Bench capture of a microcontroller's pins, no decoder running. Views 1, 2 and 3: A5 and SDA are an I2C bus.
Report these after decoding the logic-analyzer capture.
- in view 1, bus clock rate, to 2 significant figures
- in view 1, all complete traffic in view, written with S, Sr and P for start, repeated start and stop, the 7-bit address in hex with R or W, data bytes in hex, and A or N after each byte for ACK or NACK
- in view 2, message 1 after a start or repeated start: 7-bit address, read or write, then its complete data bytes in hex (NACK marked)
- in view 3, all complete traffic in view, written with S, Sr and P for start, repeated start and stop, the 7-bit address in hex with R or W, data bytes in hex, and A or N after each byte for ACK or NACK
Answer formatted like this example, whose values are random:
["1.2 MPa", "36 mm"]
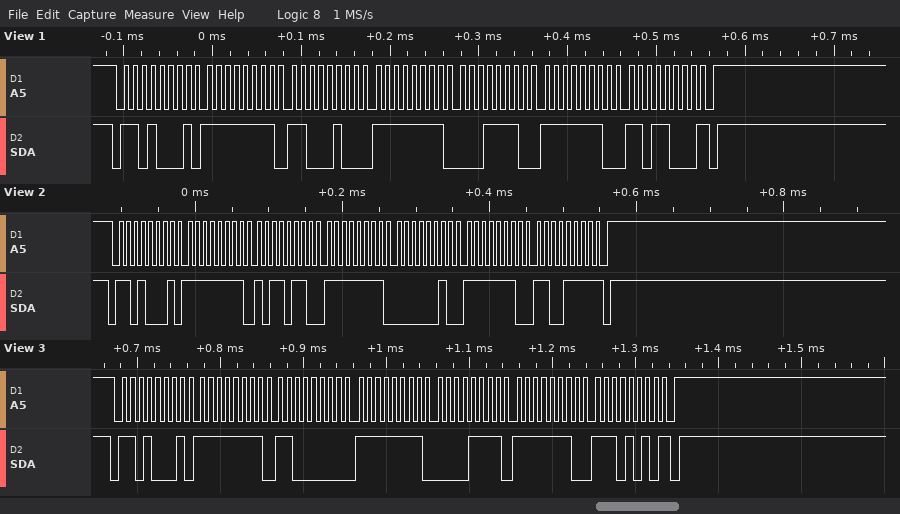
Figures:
["100 kHz", "S 68R A FF A C4 A FF A 1E A FE A D8 N P", "0x68 read: FF B6 FF 02 FE CF NACK", "S 68R A FF A C0 A FF A 0F A FE A EA N P"]
